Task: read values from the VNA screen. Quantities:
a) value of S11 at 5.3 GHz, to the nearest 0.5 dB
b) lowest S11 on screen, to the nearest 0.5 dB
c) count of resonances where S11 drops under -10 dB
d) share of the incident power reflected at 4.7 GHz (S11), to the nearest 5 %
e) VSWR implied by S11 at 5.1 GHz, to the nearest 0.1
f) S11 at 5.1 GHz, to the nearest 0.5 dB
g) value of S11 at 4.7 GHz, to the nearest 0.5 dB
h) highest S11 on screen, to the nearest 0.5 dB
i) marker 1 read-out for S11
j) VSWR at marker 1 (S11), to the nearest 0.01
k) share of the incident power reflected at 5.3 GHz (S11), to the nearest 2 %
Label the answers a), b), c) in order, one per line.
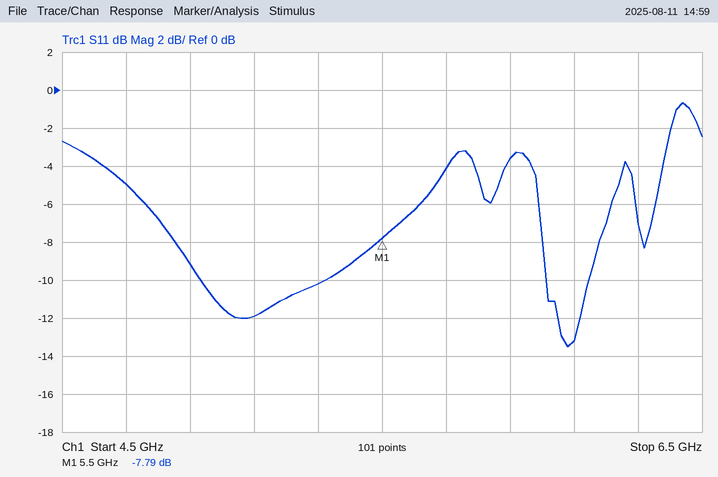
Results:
a) -10.0 dB
b) -13.5 dB
c) 2
d) 30 %
e) 1.7
f) -12.0 dB
g) -5.0 dB
h) -0.5 dB
i) -7.79 dB
j) 2.38
k) 10 %
